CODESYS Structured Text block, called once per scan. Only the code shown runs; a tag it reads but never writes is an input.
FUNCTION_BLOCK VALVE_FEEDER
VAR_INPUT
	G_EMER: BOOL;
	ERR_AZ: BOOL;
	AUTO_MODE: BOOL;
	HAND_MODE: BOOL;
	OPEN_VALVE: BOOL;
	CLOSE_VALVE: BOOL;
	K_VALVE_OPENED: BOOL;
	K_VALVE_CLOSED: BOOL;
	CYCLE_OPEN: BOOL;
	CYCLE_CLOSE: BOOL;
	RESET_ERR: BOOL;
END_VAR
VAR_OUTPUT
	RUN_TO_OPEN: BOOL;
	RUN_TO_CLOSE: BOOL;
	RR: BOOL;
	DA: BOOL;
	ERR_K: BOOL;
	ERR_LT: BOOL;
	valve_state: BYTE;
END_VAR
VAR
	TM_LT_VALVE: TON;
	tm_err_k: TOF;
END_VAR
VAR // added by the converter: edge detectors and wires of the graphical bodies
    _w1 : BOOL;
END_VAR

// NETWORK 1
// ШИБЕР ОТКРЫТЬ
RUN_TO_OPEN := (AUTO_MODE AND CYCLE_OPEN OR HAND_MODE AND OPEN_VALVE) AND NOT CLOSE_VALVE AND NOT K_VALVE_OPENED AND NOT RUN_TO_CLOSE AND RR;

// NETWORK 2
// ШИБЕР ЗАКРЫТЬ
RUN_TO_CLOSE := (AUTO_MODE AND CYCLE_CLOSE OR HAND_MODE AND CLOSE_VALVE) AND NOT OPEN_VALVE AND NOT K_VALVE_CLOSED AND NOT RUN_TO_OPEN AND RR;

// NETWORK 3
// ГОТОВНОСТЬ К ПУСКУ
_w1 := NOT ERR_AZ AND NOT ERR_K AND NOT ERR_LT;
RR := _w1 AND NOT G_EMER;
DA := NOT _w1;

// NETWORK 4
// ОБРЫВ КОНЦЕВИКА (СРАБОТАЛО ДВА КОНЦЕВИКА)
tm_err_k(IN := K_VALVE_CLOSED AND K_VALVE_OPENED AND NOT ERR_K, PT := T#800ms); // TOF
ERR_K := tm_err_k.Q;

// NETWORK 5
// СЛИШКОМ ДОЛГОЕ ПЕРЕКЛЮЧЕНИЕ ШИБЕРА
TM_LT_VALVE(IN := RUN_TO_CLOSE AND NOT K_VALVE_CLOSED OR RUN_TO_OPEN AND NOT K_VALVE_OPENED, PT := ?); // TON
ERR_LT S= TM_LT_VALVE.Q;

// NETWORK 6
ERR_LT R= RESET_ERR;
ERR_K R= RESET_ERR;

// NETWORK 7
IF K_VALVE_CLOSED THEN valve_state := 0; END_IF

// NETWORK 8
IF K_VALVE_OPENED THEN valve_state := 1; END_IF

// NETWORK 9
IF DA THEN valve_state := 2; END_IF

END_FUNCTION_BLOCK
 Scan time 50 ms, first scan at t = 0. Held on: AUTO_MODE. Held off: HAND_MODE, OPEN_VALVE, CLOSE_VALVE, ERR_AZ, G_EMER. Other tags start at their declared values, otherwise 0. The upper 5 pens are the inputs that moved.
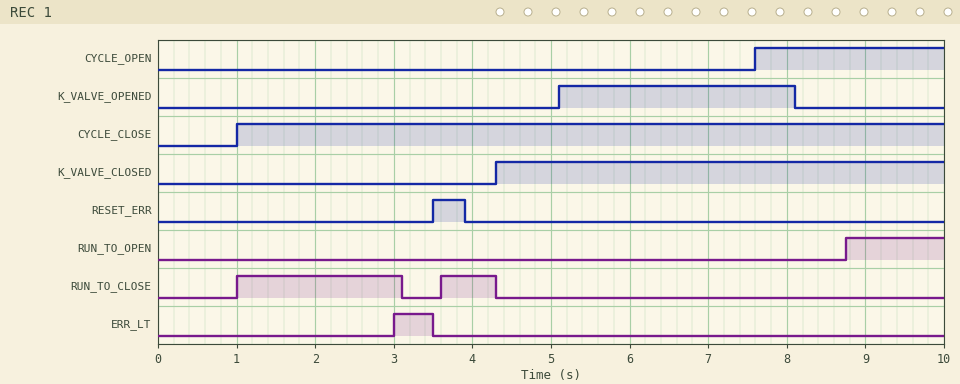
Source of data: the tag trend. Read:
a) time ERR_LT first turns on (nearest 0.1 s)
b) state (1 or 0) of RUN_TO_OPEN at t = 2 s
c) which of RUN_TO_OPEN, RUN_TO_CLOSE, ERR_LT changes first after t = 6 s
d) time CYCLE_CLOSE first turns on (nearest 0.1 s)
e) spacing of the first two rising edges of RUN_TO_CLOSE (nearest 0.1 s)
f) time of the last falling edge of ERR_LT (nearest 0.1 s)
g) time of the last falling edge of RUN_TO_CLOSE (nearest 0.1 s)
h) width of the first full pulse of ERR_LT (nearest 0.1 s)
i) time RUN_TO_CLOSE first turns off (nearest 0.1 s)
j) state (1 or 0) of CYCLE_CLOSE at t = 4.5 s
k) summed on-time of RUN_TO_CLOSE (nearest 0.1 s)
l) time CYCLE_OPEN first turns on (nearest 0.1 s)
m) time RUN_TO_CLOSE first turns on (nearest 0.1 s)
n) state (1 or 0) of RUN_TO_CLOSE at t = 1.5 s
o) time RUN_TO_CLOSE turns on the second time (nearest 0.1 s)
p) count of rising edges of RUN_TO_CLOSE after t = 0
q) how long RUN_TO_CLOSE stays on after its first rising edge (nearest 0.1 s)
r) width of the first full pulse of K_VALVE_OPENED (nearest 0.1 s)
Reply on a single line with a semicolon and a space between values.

3.0 s; 0; RUN_TO_OPEN; 1.0 s; 2.6 s; 3.5 s; 4.3 s; 0.5 s; 3.1 s; 1; 2.8 s; 7.6 s; 1.0 s; 1; 3.6 s; 2; 2.1 s; 3.0 s
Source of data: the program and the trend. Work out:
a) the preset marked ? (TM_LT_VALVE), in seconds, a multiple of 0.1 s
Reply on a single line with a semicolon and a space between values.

2.0 s
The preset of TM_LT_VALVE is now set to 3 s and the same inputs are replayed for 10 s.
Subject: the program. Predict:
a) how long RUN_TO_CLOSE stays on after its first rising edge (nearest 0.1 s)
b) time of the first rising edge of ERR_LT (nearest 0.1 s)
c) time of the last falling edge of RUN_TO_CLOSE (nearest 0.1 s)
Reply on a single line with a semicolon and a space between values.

3.1 s; 4.0 s; 4.1 s
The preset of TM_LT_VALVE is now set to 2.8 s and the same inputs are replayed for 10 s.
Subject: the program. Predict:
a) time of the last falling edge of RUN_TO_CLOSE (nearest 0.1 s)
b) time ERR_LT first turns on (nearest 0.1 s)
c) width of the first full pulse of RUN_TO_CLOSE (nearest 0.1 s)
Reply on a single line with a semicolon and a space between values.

4.0 s; 3.9 s; 3.0 s
